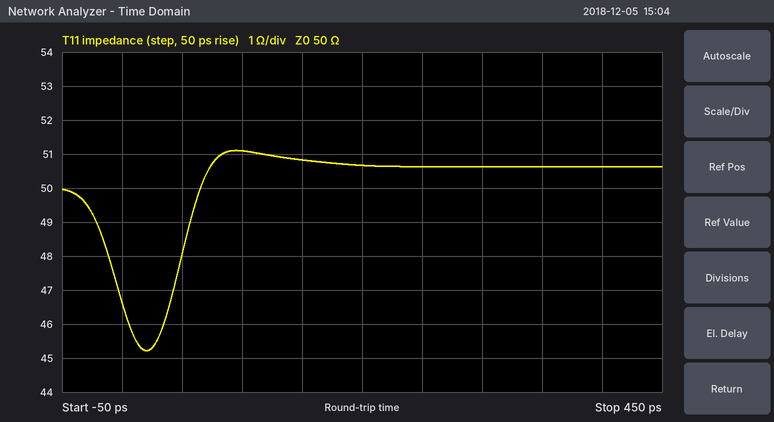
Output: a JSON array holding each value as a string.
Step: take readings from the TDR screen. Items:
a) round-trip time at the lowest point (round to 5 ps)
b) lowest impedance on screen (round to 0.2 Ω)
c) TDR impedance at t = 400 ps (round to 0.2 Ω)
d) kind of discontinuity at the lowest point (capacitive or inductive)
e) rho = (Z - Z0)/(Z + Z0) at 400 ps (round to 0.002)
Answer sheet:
["20 ps", "45.2 Ω", "50.6 Ω", "capacitive", "+0.006"]
